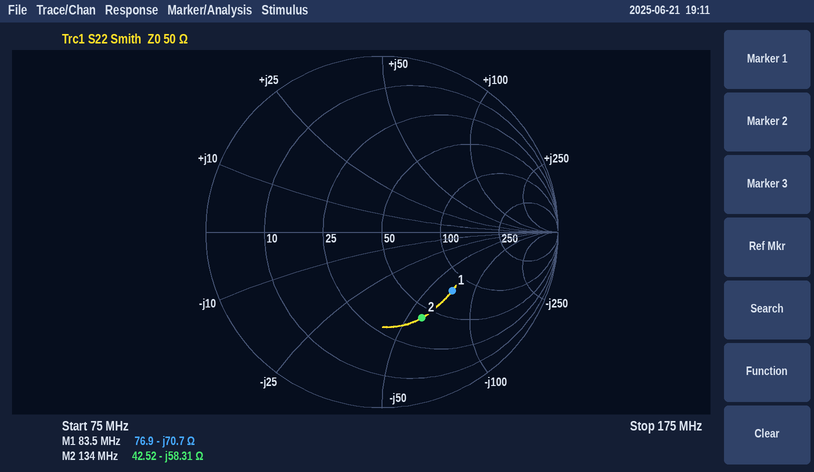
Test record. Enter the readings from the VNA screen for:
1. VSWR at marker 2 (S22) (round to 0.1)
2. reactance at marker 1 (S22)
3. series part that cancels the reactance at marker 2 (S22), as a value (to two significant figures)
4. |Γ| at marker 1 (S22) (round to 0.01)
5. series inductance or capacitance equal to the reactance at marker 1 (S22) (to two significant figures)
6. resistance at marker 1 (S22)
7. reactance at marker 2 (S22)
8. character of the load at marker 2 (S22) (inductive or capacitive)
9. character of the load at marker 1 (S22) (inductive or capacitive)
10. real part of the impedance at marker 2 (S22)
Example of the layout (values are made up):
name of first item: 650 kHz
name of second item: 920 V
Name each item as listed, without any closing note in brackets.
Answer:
VSWR at marker 2 (S22): 3.3
reactance at marker 1: -70.7 Ω
series part that cancels the reactance at marker 2 (S22), as a value: 69 nH
|Γ| at marker 1 (S22): 0.52
series inductance or capacitance equal to the reactance at marker 1 (S22): 27 pF
resistance at marker 1: 76.9 Ω
reactance at marker 2: -58.31 Ω
character of the load at marker 2 (S22): capacitive
character of the load at marker 1 (S22): capacitive
real part of the impedance at marker 2: 42.52 Ω
